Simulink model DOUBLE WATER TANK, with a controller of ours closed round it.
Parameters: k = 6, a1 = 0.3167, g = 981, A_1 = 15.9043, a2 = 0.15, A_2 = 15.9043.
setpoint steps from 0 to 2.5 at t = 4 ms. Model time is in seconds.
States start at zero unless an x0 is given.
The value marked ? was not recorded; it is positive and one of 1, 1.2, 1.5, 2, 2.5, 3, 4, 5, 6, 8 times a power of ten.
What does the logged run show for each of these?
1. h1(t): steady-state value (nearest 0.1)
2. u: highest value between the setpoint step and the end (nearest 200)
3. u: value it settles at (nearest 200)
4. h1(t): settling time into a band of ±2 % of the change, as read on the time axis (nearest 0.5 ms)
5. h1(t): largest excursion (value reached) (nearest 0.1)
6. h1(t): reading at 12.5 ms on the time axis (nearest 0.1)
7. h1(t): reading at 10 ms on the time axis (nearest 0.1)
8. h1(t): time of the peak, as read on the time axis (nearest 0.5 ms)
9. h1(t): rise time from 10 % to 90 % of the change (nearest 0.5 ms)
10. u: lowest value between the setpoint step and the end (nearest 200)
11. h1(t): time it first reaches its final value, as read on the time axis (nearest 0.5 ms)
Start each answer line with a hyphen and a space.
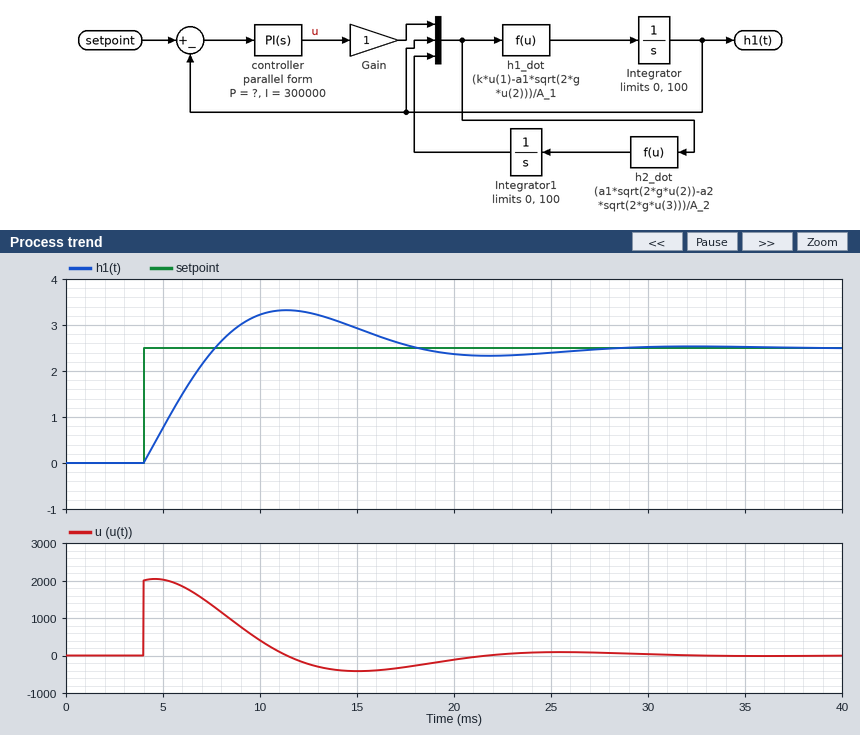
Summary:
- 2.5
- 2000
- 0
- 26.5 ms
- 3.3
- 3.3
- 3.2
- 11.5 ms
- 3.0 ms
- -400
- 7.5 ms
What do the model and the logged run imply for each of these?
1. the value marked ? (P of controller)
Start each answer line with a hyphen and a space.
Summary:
- 800
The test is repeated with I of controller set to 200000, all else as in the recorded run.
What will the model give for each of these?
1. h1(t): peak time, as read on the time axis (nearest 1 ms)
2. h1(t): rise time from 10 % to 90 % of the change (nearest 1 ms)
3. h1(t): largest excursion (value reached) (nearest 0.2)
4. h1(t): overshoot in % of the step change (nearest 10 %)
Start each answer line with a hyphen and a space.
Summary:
- 13 ms
- 3 ms
- 3.2
- 30 %
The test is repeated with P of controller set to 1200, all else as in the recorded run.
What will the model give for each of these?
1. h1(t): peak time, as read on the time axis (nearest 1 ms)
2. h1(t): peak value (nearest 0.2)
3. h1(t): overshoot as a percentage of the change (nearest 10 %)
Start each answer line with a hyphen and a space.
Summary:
- 11 ms
- 3.0
- 20 %
